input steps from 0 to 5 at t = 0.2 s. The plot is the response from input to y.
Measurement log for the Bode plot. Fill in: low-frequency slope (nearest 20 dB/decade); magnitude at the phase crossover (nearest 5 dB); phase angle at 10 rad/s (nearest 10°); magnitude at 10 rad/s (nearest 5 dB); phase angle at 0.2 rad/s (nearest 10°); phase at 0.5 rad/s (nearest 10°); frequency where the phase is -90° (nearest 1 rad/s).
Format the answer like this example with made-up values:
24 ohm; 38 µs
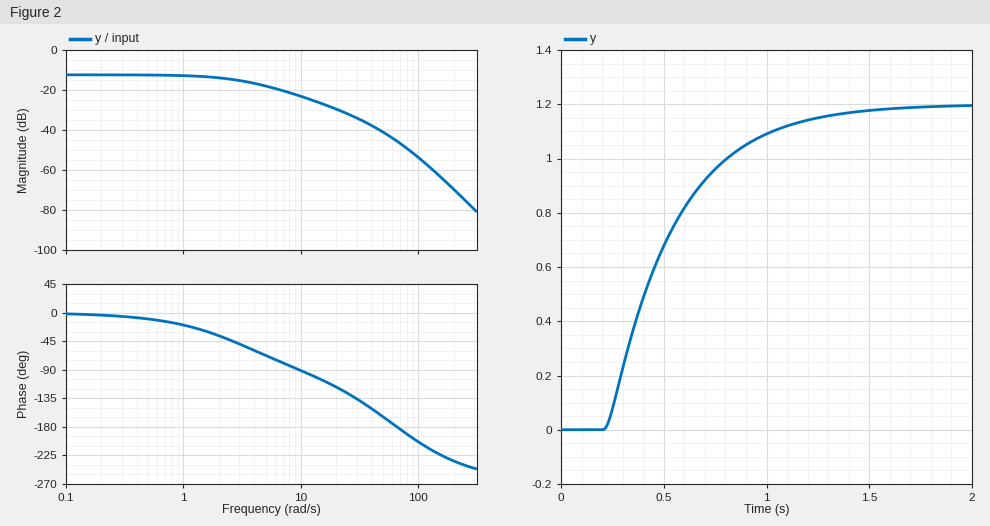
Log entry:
0 dB/decade; -45 dB; -90°; -25 dB; 0°; -10°; 10 rad/s
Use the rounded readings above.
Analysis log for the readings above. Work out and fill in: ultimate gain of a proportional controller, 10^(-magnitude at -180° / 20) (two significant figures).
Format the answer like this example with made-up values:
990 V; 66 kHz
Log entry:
180
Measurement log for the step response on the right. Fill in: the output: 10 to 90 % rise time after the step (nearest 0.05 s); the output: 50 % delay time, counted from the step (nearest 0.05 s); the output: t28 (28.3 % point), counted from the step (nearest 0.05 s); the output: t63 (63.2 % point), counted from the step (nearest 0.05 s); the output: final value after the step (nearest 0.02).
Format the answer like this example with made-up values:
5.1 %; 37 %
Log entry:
0.70 s; 0.25 s; 0.15 s; 0.35 s; 1.20
